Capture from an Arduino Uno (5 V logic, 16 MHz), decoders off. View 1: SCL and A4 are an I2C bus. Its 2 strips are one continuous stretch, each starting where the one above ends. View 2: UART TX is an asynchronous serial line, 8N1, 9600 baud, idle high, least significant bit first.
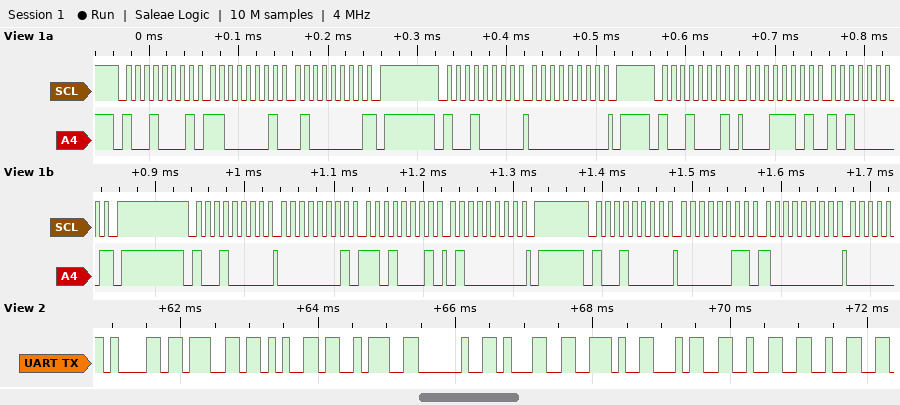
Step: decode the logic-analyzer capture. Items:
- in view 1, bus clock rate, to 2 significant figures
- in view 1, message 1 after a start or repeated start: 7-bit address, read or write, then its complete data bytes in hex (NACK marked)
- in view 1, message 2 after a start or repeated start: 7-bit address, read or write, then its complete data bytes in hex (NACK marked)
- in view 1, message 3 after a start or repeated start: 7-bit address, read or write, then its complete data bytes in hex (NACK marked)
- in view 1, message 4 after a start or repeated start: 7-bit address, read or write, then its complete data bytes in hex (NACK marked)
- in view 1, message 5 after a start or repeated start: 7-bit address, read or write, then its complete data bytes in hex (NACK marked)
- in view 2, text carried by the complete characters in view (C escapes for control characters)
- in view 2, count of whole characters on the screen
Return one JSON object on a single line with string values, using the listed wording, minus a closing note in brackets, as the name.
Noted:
{"in view 1, bus clock rate, to 2 significant figures": "100 kHz", "in view 1, message 1 after a start or repeated start: 7-bit address, read or write, then its complete data bytes in hex": "0x48 read: C1 40 NACK", "in view 1, message 2 after a start or repeated start: 7-bit address, read or write, then its complete data bytes in hex": "0x48 write: 00", "in view 1, message 3 after a start or repeated start: 7-bit address, read or write, then its complete data bytes in hex": "0x48 read: 1D A0 NACK", "in view 1, message 4 after a start or repeated start: 7-bit address, read or write, then its complete data bytes in hex": "0x48 write: 01 D1 40", "in view 1, message 5 after a start or repeated start: 7-bit address, read or write, then its complete data bytes in hex": "0x48 write: 03 80", "in view 2, text carried by the complete characters in view": "\"age: 1.422\"", "in view 2, count of whole characters on the screen": "10"}
